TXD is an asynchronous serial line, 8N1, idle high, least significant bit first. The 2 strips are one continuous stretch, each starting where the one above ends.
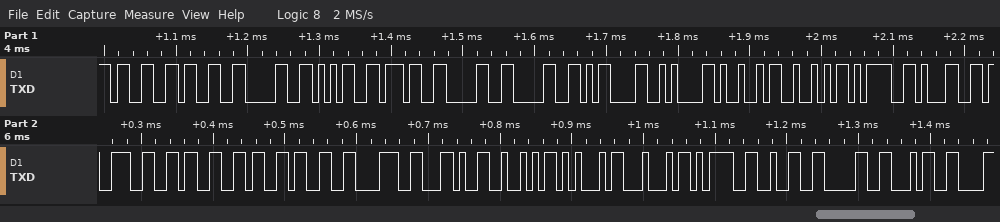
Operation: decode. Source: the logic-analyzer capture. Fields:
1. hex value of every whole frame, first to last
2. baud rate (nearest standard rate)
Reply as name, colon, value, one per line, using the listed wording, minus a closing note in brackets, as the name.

hex value of every whole frame, first to last: 33 33 30 35 37 30 30 0D 0A 49 52 3D 31 39 36 36 33 38 2C 52 45 44 3D 32 30 34
baud rate: 115200 baud
